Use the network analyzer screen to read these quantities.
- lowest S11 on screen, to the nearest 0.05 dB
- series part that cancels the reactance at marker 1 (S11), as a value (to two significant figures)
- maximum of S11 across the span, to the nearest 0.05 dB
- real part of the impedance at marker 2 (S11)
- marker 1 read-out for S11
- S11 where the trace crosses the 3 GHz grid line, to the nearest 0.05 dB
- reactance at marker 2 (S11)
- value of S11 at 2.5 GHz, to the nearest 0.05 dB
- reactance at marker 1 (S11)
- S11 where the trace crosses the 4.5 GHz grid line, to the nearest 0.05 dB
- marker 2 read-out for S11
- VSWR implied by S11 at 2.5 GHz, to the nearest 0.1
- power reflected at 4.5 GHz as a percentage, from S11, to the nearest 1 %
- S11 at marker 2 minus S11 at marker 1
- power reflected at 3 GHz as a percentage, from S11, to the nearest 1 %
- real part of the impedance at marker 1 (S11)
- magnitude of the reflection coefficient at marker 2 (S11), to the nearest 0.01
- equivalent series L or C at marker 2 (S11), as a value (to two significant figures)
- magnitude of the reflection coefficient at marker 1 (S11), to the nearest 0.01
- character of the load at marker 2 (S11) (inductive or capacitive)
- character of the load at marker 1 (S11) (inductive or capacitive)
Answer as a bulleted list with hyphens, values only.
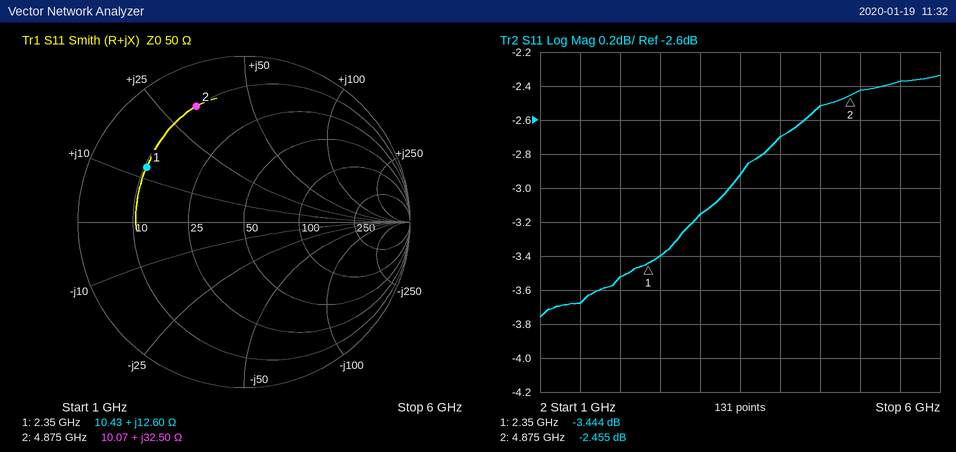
- -3.75 dB
- 5.4 pF
- -2.35 dB
- 10.07 Ω
- -3.444 dB
- -3.15 dB
- +32.50 Ω
- -3.40 dB
- +12.60 Ω
- -2.50 dB
- -2.455 dB
- 5.2
- 56 %
- 0.989 dB
- 48 %
- 10.43 Ω
- 0.75
- 1.1 nH
- 0.67
- inductive
- inductive
